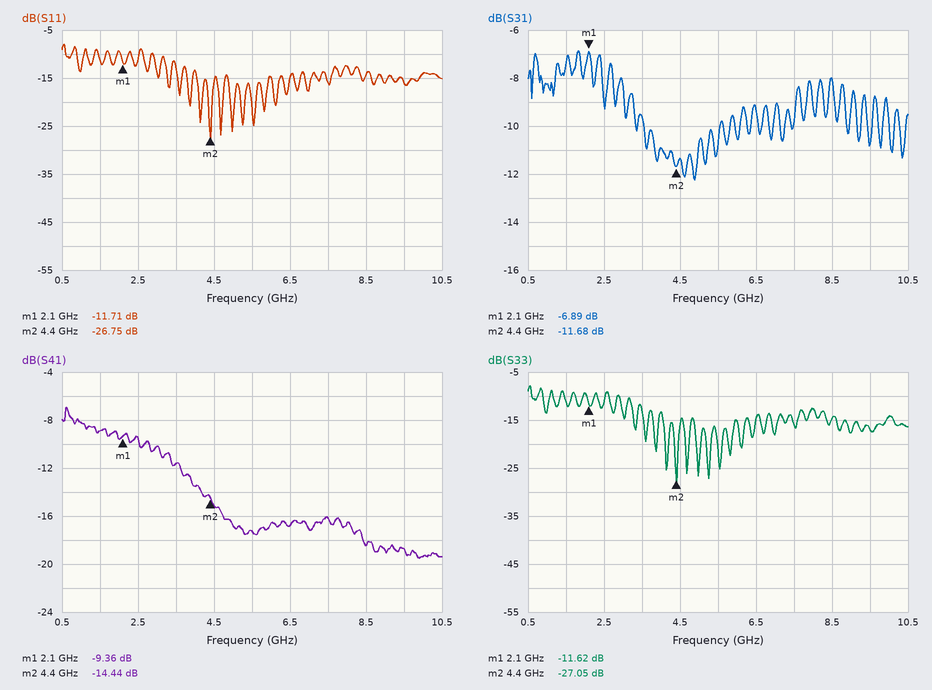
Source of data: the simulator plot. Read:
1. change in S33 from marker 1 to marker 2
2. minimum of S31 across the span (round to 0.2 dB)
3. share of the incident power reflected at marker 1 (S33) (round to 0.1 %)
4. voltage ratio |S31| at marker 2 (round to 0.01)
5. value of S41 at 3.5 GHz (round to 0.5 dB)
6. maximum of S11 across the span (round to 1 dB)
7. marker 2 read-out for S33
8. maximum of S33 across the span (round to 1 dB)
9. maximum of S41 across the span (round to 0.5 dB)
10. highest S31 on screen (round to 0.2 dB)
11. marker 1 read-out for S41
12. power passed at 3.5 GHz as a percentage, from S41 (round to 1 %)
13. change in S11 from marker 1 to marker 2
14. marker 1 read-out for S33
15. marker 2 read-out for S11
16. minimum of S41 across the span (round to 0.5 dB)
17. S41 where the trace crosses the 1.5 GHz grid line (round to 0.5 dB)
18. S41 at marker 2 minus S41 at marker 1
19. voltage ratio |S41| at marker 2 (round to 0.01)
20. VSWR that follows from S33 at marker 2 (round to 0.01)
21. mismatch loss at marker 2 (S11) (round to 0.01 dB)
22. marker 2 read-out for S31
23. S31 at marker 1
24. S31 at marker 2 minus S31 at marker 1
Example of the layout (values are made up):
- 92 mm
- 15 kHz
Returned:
- -15.43 dB
- -12.2 dB
- 6.9 %
- 0.26
- -11.5 dB
- -8 dB
- -27.05 dB
- -8 dB
- -7.0 dB
- -6.8 dB
- -9.36 dB
- 7 %
- -15.04 dB
- -11.62 dB
- -26.75 dB
- -19.5 dB
- -9.0 dB
- -5.08 dB
- 0.19
- 1.09
- 0.01 dB
- -11.68 dB
- -6.89 dB
- -4.79 dB
